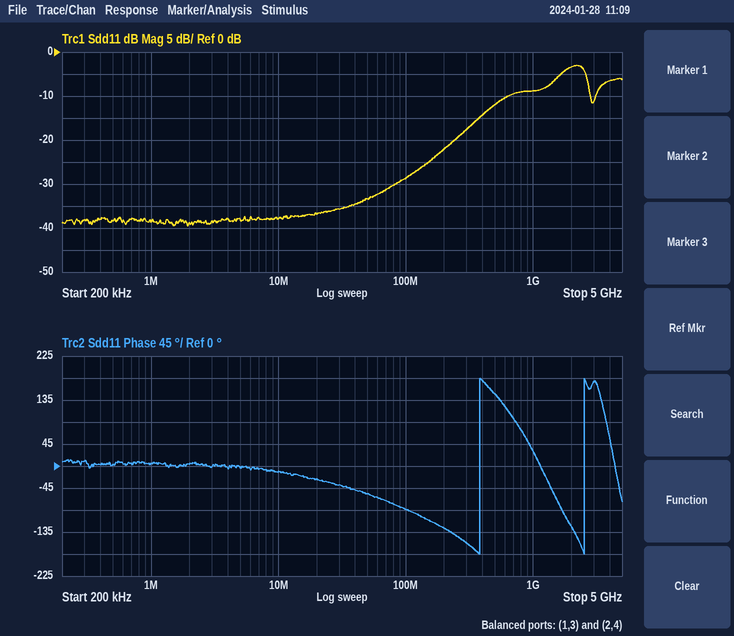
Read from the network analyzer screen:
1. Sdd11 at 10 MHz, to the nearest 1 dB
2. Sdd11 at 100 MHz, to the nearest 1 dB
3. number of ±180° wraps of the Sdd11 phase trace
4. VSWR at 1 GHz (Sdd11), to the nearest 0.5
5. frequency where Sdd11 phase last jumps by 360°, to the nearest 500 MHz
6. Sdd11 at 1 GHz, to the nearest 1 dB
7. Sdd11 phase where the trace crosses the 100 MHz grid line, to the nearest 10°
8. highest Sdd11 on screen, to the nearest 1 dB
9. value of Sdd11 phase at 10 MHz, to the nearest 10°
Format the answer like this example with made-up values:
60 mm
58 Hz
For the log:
-38 dB
-29 dB
2
2.0
2.5 GHz
-9 dB
-90°
-3 dB
-10°
